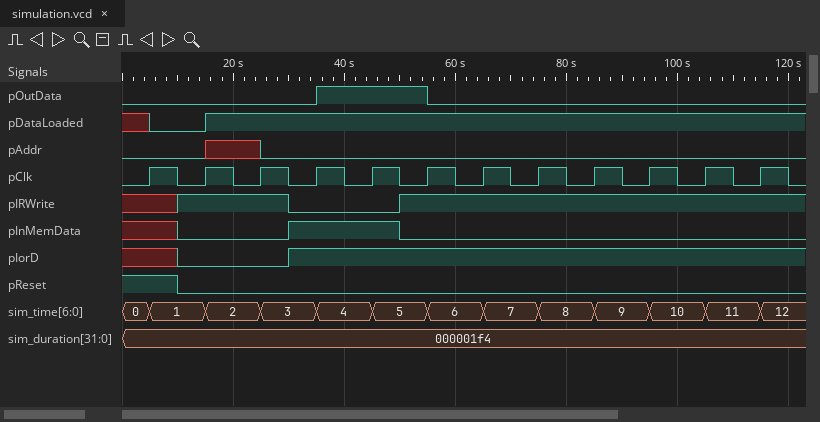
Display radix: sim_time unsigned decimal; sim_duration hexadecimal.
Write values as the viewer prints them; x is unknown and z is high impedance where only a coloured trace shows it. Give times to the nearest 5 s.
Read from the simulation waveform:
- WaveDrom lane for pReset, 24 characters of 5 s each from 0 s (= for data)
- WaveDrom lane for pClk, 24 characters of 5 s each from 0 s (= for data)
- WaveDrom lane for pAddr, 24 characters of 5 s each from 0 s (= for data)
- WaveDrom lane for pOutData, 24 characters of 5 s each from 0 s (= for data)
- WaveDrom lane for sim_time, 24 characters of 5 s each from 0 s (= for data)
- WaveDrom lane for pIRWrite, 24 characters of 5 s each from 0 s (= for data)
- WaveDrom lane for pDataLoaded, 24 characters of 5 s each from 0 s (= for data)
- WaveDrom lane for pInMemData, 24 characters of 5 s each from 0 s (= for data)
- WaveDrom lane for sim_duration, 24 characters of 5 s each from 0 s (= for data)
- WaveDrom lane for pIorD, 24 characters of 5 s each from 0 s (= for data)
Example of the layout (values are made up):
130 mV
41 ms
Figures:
{name: 'pReset', wave: '1.0.....................'}
{name: 'pClk', wave: '010101010101010101010101'}
{name: 'pAddr', wave: '0..x.0..................'}
{name: 'pOutData', wave: '0......1...0............'}
{name: 'sim_time', wave: '==.=.=.=.=.=.=.=.=.=.=.=', data: '0 1 2 3 4 5 6 7 8 9 10 11 12'}
{name: 'pIRWrite', wave: 'x.1...0...1.............'}
{name: 'pDataLoaded', wave: 'x0.1....................'}
{name: 'pInMemData', wave: 'x.0...1...0.............'}
{name: 'sim_duration', wave: '=.......................', data: '000001f4'}
{name: 'pIorD', wave: 'x.0...1.................'}
